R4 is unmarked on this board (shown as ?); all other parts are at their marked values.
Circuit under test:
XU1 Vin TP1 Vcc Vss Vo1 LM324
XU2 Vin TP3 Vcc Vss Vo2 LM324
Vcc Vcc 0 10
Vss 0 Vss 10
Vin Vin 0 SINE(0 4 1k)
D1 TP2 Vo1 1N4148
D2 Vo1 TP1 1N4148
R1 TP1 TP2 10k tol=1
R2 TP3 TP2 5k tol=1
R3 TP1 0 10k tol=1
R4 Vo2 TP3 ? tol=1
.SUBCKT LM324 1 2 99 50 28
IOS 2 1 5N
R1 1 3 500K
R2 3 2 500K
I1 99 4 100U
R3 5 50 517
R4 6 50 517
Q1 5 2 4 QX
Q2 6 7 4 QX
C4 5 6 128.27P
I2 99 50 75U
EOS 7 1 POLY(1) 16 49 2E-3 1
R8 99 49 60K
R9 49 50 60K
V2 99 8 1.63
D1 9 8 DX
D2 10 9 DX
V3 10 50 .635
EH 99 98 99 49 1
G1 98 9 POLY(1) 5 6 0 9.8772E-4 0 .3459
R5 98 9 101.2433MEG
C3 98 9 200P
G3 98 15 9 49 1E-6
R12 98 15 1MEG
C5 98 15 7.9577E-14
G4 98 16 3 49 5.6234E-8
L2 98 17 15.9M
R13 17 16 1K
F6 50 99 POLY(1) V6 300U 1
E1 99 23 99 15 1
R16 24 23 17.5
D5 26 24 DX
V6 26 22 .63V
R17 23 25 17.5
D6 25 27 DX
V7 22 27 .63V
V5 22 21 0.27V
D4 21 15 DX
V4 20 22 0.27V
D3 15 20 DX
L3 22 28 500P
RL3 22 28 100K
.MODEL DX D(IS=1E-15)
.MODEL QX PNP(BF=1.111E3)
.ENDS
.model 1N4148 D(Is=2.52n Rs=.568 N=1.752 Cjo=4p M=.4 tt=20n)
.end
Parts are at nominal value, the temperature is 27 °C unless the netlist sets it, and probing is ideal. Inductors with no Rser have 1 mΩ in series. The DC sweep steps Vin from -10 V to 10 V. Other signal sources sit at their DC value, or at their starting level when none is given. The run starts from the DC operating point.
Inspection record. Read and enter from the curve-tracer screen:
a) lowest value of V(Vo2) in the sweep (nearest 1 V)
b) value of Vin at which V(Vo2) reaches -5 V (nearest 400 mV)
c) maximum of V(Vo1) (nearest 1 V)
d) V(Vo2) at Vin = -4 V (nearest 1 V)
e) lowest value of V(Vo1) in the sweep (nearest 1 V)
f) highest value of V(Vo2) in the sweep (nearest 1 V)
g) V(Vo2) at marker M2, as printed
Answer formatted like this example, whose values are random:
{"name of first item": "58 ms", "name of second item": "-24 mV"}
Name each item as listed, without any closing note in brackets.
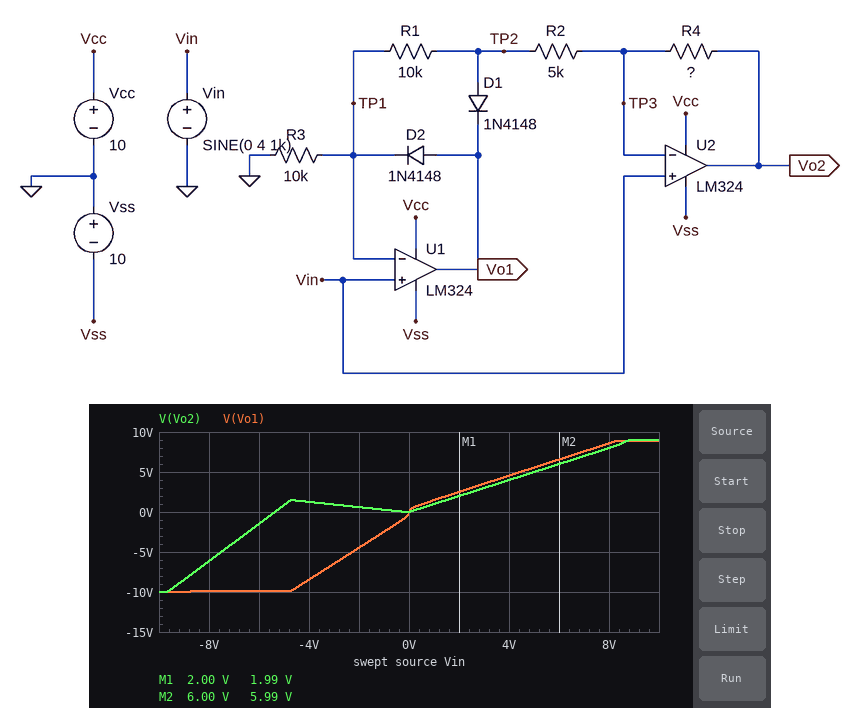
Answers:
{"lowest value of V(Vo2) in the sweep": "-10 V", "value of Vin at which V(Vo2) reaches -5 V": "-7.6 V", "maximum of V(Vo1)": "9 V", "V(Vo2) at Vin = -4 V": "1 V", "lowest value of V(Vo1) in the sweep": "-10 V", "highest value of V(Vo2) in the sweep": "9 V", "V(Vo2) at marker M2, as printed": "5.99 V"}
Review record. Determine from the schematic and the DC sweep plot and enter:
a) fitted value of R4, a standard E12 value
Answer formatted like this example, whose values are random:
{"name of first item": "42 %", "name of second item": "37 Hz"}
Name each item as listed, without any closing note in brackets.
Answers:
{"fitted value of R4, a standard E12 value": "6.8 kΩ"}
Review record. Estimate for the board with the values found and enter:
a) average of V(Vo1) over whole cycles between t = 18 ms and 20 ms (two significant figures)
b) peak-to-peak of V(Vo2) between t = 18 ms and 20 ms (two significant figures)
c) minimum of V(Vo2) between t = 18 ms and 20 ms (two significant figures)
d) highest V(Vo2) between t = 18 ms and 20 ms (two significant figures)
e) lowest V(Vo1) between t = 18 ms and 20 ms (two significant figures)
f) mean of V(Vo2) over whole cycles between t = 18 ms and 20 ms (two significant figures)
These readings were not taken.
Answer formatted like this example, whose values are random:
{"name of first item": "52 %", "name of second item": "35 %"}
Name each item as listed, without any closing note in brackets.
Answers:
{"average of V(Vo1) over whole cycles between t = 18 ms and 20 ms": "-1.3 V", "peak-to-peak of V(Vo2) between t = 18 ms and 20 ms": "4.1 V", "minimum of V(Vo2) between t = 18 ms and 20 ms": "-120 mV", "highest V(Vo2) between t = 18 ms and 20 ms": "4.0 V", "lowest V(Vo1) between t = 18 ms and 20 ms": "-8.6 V", "mean of V(Vo2) over whole cycles between t = 18 ms and 20 ms": "1.7 V"}
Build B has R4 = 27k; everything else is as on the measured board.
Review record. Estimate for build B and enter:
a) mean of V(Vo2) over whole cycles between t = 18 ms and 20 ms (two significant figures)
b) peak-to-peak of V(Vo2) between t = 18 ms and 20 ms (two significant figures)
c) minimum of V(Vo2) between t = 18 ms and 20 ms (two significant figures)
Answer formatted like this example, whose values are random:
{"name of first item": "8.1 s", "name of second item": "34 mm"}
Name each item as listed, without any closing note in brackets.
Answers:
{"mean of V(Vo2) over whole cycles between t = 18 ms and 20 ms": "5.0 V", "peak-to-peak of V(Vo2) between t = 18 ms and 20 ms": "9.1 V", "minimum of V(Vo2) between t = 18 ms and 20 ms": "-160 mV"}
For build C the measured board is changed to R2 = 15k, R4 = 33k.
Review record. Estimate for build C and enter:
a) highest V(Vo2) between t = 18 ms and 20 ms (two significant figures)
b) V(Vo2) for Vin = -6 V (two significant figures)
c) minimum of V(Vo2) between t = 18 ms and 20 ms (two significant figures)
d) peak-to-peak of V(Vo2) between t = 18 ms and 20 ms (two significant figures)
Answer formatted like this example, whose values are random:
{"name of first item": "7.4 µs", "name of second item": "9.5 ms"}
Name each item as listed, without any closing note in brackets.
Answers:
{"highest V(Vo2) between t = 18 ms and 20 ms": "4.8 V", "V(Vo2) for Vin = -6 V": "1.4 V", "minimum of V(Vo2) between t = 18 ms and 20 ms": "-140 mV", "peak-to-peak of V(Vo2) between t = 18 ms and 20 ms": "4.9 V"}
